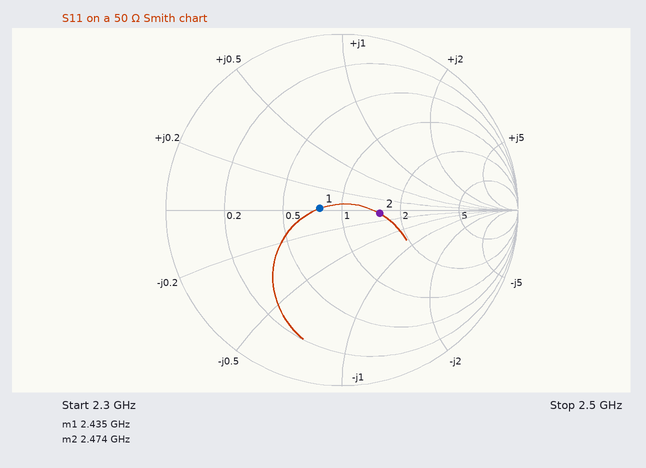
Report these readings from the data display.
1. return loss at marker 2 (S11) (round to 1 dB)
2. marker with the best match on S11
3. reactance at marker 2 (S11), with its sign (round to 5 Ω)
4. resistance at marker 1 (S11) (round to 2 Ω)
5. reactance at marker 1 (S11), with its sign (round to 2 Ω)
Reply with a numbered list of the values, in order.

1. 13 dB
2. marker 1
3. -5 Ω
4. 38 Ω
5. 0 Ω
